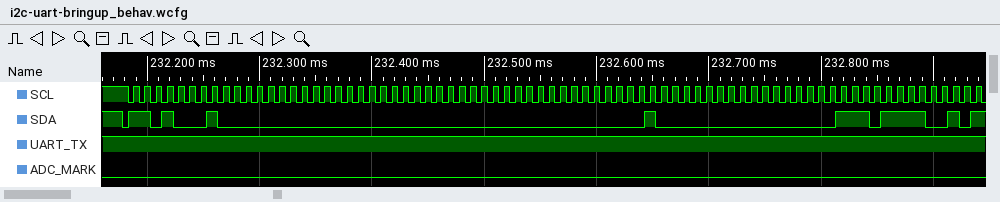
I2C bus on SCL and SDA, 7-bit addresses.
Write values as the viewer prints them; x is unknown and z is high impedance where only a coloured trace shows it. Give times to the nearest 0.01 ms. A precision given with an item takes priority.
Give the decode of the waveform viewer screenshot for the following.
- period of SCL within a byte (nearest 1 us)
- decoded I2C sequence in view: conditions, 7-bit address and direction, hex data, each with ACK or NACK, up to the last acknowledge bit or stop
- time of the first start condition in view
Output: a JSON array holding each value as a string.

["10 us", "start, address 68 read ACK, 00 ACK, 00 ACK, 00 ACK, 00 ACK, 40 ACK, 00 ACK, EF ACK", "232.18 ms"]
